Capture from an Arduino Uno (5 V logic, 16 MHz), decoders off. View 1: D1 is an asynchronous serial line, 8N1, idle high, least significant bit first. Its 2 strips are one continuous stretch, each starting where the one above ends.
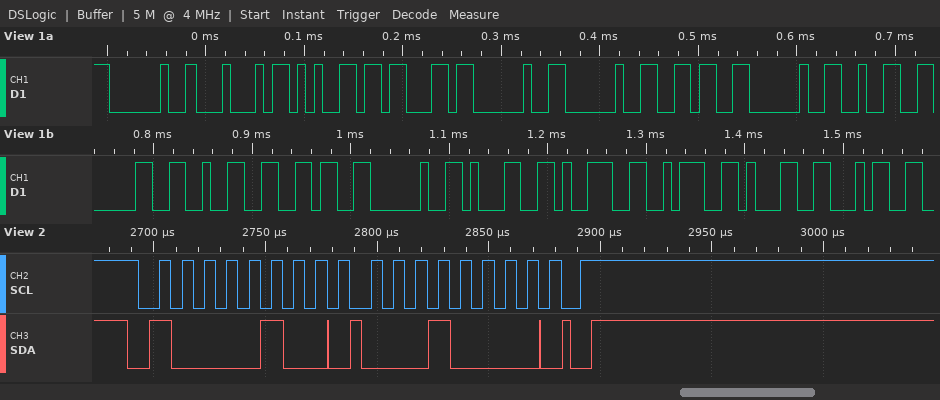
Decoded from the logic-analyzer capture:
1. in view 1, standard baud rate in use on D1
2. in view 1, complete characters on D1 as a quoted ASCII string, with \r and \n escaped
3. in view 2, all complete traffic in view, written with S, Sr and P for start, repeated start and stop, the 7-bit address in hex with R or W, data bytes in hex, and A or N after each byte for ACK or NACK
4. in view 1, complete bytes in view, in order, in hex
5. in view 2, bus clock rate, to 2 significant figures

115200 baud
" Dec  6 2026 19:14"
S 42W A 10 A P
0x20 0x44 0x65 0x63 0x20 0x20 0x36 0x20 0x32 0x30 0x32 0x36 0x20 0x31 0x39 0x3A 0x31 0x34
100 kHz
